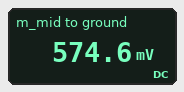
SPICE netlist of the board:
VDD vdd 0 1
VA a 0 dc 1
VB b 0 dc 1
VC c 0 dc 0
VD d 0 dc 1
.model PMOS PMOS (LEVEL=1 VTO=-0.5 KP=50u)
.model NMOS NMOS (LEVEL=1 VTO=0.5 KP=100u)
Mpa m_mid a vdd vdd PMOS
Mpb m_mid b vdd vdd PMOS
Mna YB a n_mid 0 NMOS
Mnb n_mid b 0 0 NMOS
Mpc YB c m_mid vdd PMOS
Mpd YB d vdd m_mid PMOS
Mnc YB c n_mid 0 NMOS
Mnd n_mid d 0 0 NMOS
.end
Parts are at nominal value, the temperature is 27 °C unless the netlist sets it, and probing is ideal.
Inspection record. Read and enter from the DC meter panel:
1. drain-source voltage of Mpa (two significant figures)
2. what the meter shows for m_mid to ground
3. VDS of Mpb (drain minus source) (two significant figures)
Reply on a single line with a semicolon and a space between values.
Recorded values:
-430 mV; 574.6 mV; -430 mV
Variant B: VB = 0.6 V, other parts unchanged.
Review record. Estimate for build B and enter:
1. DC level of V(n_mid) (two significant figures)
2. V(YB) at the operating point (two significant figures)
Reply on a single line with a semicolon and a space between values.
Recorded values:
2.3 mV; 5.1 mV
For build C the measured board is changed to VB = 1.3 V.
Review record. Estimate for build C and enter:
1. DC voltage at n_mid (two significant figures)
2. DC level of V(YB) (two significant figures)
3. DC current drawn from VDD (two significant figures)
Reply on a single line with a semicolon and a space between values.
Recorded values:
1.1 mV; 3.9 mV; 140 nA
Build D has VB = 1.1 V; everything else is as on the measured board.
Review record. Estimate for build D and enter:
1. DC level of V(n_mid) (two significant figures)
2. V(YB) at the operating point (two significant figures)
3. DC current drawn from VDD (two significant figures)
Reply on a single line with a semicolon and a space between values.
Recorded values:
1.3 mV; 4.1 mV; 140 nA
